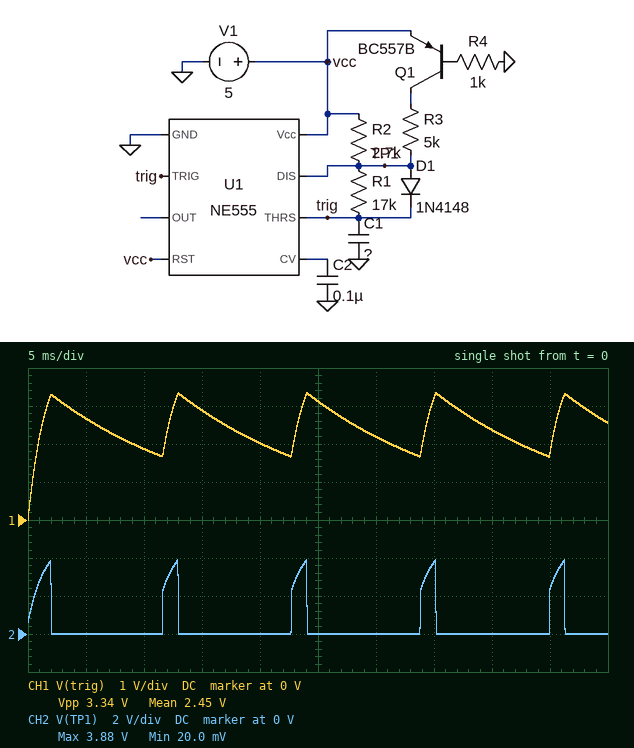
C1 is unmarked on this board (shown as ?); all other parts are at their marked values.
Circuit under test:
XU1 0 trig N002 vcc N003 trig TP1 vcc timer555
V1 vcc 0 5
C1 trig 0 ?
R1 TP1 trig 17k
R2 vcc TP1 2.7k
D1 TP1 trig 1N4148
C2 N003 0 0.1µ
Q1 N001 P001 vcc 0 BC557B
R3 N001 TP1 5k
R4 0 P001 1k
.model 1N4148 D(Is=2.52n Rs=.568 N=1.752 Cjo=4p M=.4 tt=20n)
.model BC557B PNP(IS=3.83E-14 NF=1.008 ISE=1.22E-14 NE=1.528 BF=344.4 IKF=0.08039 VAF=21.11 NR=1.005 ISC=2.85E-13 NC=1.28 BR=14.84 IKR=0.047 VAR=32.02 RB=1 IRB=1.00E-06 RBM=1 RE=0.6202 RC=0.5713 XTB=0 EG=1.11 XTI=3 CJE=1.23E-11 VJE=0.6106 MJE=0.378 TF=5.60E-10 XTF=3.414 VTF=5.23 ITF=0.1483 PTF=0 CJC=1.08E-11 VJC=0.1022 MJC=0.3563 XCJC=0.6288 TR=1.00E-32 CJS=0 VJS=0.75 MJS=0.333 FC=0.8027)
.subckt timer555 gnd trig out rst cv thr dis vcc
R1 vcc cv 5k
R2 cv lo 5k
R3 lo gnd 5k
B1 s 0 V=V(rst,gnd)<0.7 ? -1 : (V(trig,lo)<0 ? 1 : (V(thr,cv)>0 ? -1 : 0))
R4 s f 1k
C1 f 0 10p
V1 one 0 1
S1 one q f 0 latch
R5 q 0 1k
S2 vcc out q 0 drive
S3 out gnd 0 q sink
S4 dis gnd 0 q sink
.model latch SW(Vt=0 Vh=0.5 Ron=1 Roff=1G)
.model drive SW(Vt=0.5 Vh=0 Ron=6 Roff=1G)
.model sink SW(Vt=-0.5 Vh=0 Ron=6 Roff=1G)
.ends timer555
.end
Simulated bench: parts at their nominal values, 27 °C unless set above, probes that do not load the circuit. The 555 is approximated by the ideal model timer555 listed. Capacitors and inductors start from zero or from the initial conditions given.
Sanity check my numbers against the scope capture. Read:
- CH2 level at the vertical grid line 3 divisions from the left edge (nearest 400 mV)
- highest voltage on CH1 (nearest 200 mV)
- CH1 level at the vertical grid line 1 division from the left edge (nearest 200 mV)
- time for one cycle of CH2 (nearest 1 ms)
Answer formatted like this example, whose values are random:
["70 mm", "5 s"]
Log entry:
["0 V", "3.4 V", "2.6 V", "11 ms"]
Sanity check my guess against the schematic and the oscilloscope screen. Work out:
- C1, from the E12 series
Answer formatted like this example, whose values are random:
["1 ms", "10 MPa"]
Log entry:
["820 nF"]
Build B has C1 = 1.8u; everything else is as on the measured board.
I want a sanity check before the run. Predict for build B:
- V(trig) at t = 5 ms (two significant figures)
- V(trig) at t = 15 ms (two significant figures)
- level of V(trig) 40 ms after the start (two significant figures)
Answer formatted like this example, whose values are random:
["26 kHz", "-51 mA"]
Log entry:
["3.3 V", "2.4 V", "2.3 V"]
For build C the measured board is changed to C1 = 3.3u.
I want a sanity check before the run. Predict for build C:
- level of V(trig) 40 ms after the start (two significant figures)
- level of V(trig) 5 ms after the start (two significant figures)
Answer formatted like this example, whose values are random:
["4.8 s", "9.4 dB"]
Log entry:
["1.9 V", "2.5 V"]
